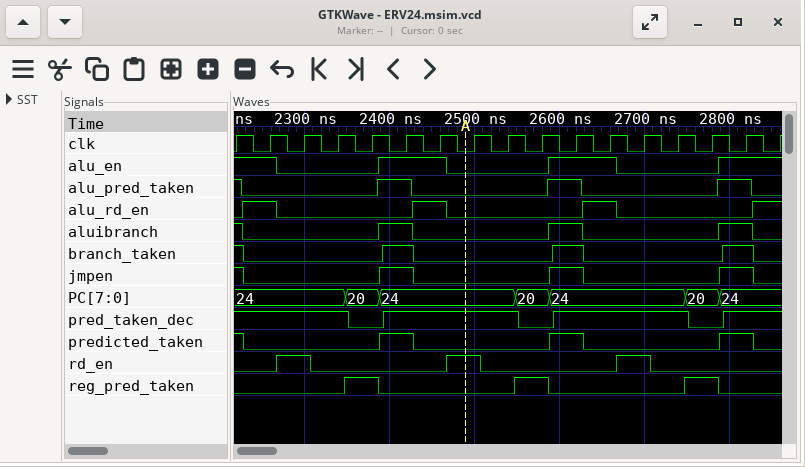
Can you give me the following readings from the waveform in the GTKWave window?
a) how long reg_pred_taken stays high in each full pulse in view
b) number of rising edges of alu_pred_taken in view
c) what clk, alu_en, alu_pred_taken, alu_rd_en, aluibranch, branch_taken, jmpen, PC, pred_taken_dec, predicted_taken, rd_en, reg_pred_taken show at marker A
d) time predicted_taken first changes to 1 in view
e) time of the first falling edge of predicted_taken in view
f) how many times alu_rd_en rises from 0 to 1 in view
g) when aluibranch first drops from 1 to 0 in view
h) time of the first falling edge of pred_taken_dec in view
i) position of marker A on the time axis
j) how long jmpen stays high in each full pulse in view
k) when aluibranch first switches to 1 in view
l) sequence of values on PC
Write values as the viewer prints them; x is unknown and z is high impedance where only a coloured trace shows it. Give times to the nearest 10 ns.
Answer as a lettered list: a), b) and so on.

a) 40 ns, 40 ns, 40 ns
b) 3
c) clk=0, alu_en=0, alu_pred_taken=0, alu_rd_en=0, aluibranch=0, branch_taken=0, jmpen=0, PC=24, pred_taken_dec=1, predicted_taken=0, rd_en=1, reg_pred_taken=0
d) 2390 ns
e) 2230 ns
f) 4
g) 2230 ns
h) 2350 ns
i) 2490 ns
j) 40 ns, 40 ns, 40 ns
k) 2390 ns
l) 24, 20, 24, 20, 24, 20, 24
